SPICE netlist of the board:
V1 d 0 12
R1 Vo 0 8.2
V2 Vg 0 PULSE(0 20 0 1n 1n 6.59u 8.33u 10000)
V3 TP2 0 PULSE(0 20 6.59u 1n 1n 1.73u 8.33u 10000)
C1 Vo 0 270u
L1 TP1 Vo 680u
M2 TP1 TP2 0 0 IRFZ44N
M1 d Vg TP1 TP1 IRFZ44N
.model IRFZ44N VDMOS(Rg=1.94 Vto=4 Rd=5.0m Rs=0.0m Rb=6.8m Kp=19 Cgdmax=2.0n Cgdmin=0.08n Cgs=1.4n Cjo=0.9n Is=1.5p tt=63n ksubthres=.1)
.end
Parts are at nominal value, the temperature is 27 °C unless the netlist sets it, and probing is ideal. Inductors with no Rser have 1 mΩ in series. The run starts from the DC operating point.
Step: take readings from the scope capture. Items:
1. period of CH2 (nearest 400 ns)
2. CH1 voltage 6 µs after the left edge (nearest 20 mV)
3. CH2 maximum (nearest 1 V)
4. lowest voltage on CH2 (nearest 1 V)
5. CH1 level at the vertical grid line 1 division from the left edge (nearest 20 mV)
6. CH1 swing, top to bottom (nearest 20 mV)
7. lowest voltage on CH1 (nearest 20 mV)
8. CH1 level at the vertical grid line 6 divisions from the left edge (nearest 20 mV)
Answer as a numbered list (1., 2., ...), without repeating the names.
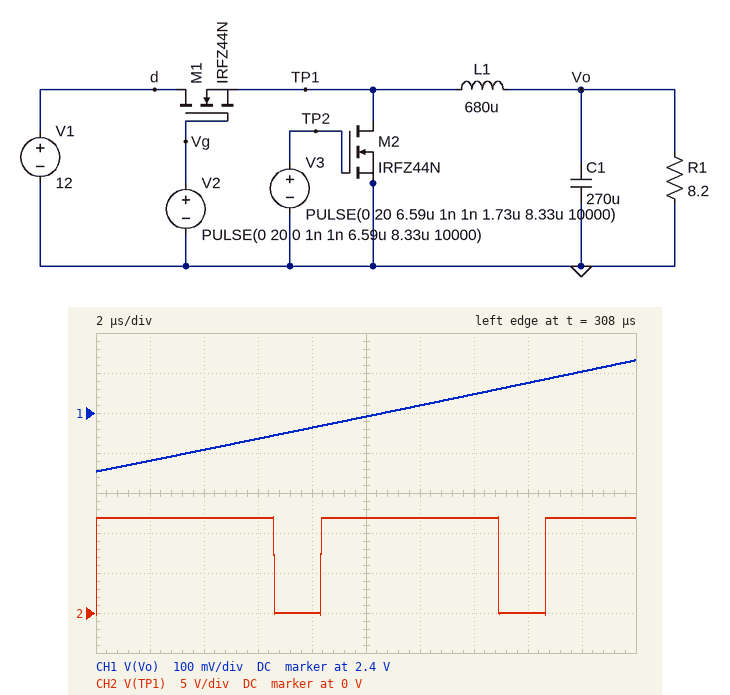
1. 8.4 µs
2. 2.34 V
3. 12 V
4. 0 V
5. 2.28 V
6. 280 mV
7. 2.26 V
8. 2.42 V
